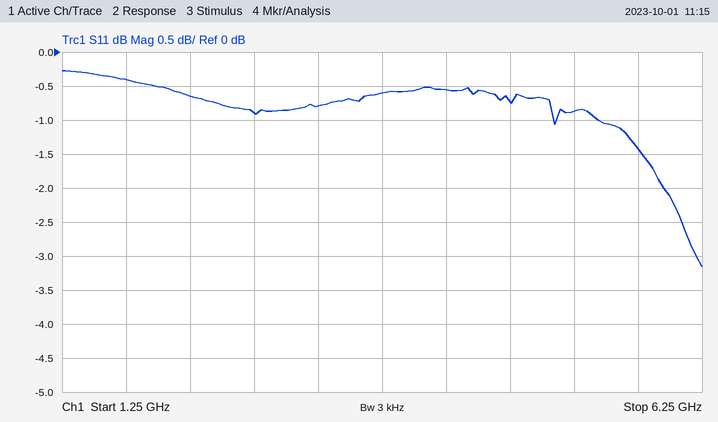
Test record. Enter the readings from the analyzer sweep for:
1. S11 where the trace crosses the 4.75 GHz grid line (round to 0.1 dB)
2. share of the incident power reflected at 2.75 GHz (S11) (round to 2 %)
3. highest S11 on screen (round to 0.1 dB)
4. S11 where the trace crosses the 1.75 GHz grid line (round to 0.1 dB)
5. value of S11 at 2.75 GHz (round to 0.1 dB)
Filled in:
-0.7 dB
82 %
-0.3 dB
-0.4 dB
-0.9 dB
